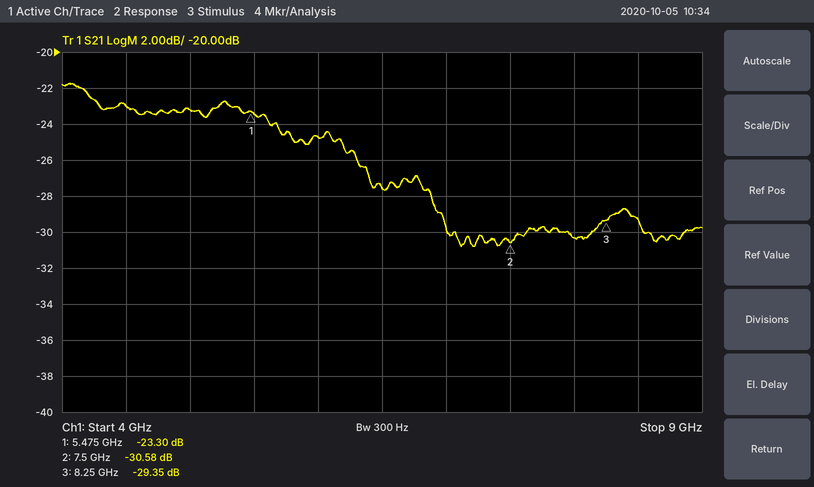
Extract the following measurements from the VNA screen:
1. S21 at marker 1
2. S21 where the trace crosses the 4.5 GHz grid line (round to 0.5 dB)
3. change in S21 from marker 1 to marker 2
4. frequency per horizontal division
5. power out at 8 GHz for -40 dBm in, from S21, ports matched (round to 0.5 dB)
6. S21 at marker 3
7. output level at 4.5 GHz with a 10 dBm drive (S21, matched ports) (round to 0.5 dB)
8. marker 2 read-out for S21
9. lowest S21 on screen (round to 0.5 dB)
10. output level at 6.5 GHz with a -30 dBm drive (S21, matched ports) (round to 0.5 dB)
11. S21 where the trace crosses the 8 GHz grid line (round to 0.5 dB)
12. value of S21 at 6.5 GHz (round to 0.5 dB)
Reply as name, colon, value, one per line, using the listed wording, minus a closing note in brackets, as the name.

S21 at marker 1: -23.30 dB
S21 where the trace crosses the 4.5 GHz grid line: -23.0 dB
change in S21 from marker 1 to marker 2: -7.28 dB
frequency per horizontal division: 500 MHz
power out at 8 GHz for -40 dBm in, from S21, ports matched: -70.5 dBm
S21 at marker 3: -29.35 dB
output level at 4.5 GHz with a 10 dBm drive (S21, matched ports): -13.0 dBm
marker 2 read-out for S21: -30.58 dB
lowest S21 on screen: -31.0 dB
output level at 6.5 GHz with a -30 dBm drive (S21, matched ports): -57.5 dBm
S21 where the trace crosses the 8 GHz grid line: -30.5 dB
value of S21 at 6.5 GHz: -27.5 dB
